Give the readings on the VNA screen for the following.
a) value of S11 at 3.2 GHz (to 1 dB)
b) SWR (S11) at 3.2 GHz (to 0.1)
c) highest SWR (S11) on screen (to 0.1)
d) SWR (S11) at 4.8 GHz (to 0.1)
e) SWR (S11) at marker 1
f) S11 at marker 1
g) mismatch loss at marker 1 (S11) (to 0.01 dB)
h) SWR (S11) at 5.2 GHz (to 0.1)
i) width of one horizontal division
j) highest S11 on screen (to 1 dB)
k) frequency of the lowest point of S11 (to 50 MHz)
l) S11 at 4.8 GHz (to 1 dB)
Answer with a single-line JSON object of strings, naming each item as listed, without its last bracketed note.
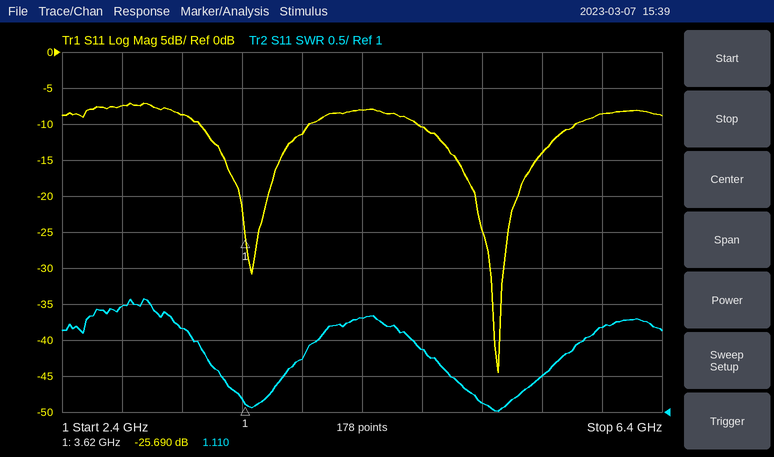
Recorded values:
{"value of S11 at 3.2 GHz": "-9 dB", "SWR (S11) at 3.2 GHz": "2.2", "highest SWR (S11) on screen": "2.6", "SWR (S11) at 4.8 GHz": "1.9", "SWR (S11) at marker 1": "1.110", "S11 at marker 1": "-25.690 dB", "mismatch loss at marker 1 (S11)": "0.01 dB", "SWR (S11) at 5.2 GHz": "1.1", "width of one horizontal division": "400 MHz", "highest S11 on screen": "-7 dB", "frequency of the lowest point of S11": "5.30 GHz", "S11 at 4.8 GHz": "-10 dB"}
